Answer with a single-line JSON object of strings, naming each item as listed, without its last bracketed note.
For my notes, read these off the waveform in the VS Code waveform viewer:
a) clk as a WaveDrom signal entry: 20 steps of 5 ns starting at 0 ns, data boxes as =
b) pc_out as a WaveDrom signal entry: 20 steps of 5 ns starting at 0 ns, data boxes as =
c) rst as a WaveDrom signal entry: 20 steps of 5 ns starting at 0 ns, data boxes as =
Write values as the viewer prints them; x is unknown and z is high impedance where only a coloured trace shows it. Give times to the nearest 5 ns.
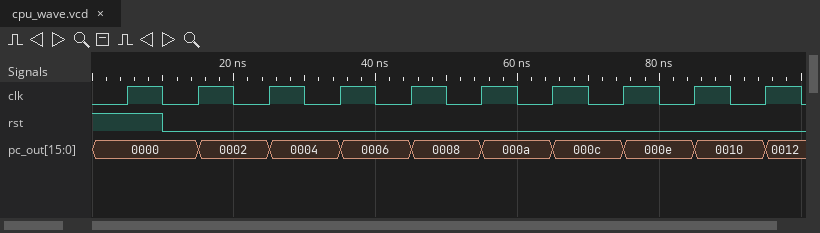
{"clk as a WaveDrom signal entry: 20 steps of 5 ns starting at 0 ns, data boxes as =": "{name: 'clk', wave: '01010101010101010101'}", "pc_out as a WaveDrom signal entry: 20 steps of 5 ns starting at 0 ns, data boxes as =": "{name: 'pc_out', wave: '=..=.=.=.=.=.=.=.=.=', data: '0000 0002 0004 0006 0008 000a 000c 000e 0010 0012'}", "rst as a WaveDrom signal entry: 20 steps of 5 ns starting at 0 ns, data boxes as =": "{name: 'rst', wave: '1.0.................'}"}
